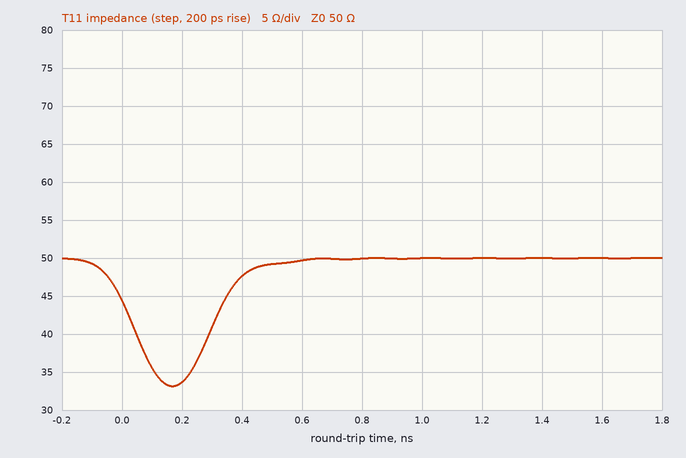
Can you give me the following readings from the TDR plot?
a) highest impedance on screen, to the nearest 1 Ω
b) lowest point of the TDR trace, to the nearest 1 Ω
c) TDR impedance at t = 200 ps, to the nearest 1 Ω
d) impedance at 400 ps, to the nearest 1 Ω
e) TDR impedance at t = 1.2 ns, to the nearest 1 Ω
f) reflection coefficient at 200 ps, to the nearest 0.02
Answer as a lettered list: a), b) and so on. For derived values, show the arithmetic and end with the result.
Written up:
a) 50 Ω
b) 33 Ω
c) 34 Ω
d) 48 Ω
e) 50 Ω
f) (34 − 50)/(34 + 50) ≈ -0.190, so -0.20 to the nearest 0.02
